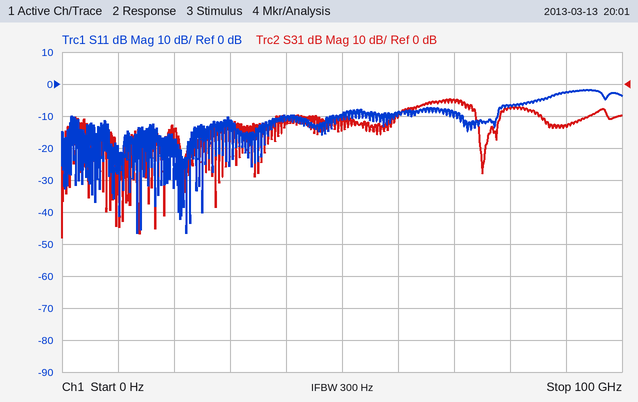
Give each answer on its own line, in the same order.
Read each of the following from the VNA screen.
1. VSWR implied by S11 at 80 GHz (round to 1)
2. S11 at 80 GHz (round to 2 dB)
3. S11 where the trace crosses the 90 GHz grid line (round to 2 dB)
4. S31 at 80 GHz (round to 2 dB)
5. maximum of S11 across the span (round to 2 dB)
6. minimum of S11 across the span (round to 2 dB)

3
-6 dB
-2 dB
-8 dB
-2 dB
-46 dB
